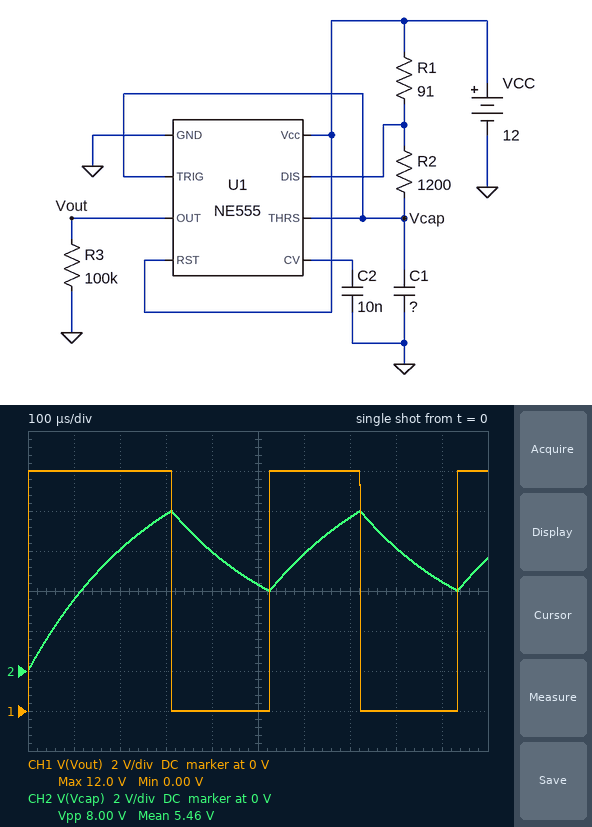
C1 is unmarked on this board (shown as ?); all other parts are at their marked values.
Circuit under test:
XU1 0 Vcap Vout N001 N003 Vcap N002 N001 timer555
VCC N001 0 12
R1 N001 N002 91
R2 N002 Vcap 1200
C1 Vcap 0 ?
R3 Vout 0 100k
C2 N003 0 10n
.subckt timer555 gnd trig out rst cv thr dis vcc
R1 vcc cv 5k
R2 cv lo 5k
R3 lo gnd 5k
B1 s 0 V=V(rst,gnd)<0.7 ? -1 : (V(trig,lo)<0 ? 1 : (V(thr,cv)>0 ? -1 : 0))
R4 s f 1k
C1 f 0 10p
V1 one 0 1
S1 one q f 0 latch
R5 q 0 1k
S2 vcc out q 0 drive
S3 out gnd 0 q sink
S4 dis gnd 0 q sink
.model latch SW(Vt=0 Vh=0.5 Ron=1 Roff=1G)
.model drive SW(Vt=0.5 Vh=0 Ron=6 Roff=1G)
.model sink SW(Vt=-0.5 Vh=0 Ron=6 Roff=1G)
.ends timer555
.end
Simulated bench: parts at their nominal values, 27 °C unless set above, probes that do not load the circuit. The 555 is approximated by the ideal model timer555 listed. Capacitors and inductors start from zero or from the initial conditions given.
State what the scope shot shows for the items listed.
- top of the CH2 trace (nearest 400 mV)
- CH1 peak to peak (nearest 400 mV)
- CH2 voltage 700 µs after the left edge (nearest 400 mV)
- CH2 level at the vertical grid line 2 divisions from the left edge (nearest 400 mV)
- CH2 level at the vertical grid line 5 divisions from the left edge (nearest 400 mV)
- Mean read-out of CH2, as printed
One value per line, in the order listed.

8.0 V
12.0 V
7.6 V
6.0 V
4.4 V
5.46 V
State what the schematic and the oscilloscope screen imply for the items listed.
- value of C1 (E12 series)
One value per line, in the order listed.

220 nF
